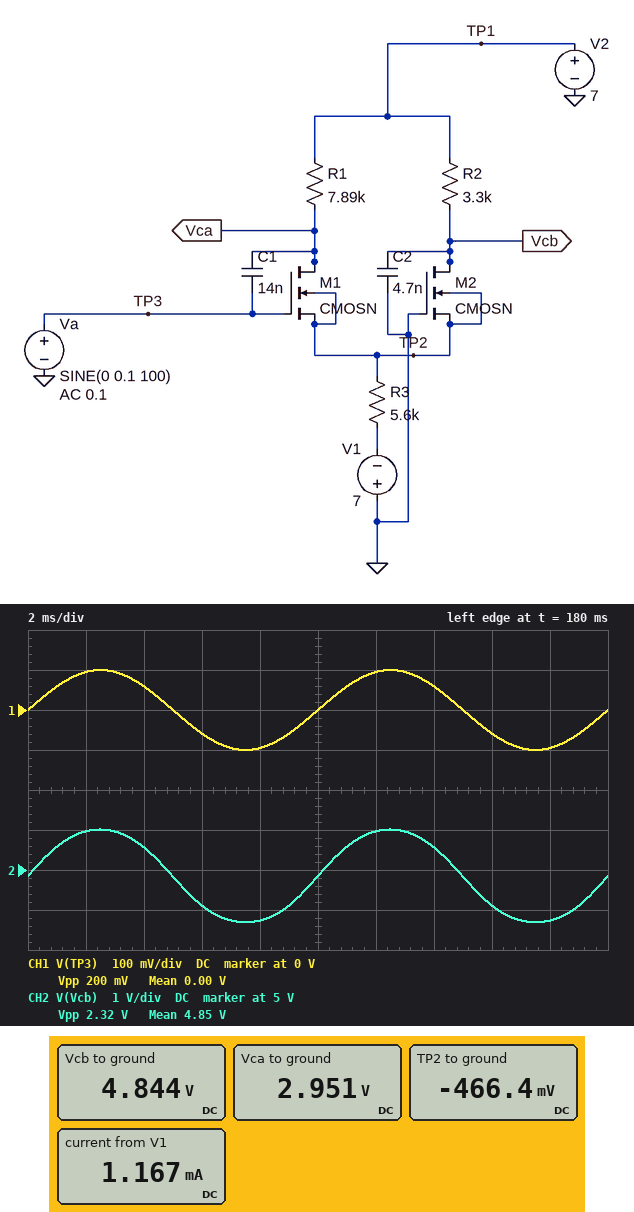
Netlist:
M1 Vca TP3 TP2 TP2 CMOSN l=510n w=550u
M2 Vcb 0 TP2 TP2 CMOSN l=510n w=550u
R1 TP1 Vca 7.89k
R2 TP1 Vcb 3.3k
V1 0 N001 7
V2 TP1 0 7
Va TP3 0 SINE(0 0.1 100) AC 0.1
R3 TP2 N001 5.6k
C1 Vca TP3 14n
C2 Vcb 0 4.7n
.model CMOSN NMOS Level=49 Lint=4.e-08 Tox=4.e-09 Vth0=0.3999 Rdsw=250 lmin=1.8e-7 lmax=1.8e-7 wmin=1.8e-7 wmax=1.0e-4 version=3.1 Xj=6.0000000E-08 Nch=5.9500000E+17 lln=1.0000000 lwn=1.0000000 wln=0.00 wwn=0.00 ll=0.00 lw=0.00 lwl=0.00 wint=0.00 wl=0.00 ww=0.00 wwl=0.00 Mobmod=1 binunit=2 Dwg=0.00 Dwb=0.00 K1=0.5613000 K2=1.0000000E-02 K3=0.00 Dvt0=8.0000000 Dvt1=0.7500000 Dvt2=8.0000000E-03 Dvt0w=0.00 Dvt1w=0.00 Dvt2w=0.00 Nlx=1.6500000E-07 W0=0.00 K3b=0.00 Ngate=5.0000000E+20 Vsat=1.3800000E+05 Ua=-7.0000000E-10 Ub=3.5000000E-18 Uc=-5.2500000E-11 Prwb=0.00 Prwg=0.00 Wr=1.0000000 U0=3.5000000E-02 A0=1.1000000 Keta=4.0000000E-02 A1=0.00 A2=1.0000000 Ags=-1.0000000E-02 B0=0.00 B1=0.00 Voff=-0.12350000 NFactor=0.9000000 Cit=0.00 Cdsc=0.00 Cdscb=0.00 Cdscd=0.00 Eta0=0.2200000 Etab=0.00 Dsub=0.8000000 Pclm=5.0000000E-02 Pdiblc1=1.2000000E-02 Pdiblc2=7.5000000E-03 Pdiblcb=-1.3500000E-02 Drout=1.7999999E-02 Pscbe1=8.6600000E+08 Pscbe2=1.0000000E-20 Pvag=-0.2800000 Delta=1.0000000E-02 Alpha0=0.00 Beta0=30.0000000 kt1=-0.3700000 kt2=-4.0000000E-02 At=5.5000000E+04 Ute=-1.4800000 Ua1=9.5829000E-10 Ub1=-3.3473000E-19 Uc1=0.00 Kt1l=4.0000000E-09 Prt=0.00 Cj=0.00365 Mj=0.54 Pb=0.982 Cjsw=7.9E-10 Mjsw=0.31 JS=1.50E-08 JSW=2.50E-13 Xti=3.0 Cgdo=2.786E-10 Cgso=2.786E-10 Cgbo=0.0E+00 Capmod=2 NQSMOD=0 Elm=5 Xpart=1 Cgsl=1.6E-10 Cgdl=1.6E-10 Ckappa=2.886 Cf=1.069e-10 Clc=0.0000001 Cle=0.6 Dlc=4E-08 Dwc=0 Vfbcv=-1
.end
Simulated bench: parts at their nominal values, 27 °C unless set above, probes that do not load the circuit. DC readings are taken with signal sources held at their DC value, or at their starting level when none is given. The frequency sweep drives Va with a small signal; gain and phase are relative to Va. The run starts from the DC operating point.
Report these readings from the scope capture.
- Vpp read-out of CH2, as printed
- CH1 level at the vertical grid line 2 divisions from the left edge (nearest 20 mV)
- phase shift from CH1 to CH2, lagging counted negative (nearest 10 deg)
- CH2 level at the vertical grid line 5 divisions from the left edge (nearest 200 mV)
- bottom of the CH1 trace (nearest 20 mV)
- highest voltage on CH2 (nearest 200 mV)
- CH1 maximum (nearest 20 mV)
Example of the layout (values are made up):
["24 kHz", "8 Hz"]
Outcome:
["2.32 V", "60 mV", "0 deg", "4.8 V", "-100 mV", "6.0 V", "100 mV"]
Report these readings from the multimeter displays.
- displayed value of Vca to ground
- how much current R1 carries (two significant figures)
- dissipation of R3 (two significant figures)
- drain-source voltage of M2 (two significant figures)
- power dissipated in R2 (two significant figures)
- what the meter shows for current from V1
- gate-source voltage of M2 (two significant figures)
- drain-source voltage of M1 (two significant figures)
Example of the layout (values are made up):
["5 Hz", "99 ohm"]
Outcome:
["2.951 V", "510 µA", "7.6 mW", "5.3 V", "1.4 mW", "1.167 mA", "470 mV", "3.4 V"]
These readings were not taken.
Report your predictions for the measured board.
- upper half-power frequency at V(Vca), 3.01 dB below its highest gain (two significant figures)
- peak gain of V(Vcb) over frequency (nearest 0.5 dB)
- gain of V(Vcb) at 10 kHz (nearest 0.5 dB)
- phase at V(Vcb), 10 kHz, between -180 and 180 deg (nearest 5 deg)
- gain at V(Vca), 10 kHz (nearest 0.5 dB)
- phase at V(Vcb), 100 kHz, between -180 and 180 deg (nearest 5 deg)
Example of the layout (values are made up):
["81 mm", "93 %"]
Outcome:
["1.9 kHz", "23.5 dB", "22.0 dB", "-40 deg", "15.5 dB", "-85 deg"]
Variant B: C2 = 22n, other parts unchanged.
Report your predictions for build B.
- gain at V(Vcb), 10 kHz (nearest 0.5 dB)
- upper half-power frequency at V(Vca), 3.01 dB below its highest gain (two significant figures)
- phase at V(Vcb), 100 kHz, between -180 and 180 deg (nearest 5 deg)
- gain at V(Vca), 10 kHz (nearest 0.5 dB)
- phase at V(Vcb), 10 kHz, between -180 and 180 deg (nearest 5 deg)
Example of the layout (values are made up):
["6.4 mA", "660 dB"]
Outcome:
["12.0 dB", "2.0 kHz", "-90 deg", "16.0 dB", "-75 deg"]
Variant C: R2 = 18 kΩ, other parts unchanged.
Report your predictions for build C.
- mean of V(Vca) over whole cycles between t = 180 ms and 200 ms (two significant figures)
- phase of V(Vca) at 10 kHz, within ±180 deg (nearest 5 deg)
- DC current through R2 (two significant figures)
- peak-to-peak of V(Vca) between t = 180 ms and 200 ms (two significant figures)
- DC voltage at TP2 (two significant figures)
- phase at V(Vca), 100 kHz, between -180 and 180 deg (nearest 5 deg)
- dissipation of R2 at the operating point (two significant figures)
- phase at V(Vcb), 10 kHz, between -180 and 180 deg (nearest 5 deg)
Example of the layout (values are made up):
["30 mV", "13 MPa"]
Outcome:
["750 mV", "70 deg", "410 µA", "1.6 V", "-500 mV", "35 deg", "3.1 mW", "-5 deg"]
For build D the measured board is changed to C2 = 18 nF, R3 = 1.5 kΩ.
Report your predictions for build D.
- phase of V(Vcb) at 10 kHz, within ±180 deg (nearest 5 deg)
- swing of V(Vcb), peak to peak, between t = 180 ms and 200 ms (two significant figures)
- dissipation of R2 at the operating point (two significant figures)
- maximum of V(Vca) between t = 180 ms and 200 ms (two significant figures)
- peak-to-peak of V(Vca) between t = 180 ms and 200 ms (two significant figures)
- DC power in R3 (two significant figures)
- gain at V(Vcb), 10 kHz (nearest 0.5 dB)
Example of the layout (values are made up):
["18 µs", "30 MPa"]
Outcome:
["30 deg", "1.6 mV", "22 mW", "-1.5 V", "1.7 mV", "20 mW", "-8.5 dB"]
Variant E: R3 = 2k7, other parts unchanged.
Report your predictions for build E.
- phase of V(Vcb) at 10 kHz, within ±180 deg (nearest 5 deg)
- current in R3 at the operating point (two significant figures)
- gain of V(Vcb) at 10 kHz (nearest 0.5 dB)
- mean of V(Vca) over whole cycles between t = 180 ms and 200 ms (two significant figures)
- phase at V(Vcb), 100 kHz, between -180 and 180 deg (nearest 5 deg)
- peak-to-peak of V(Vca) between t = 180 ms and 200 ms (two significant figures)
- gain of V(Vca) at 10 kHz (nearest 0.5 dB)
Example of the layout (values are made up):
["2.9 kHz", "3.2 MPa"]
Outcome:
["-30 deg", "2.4 mA", "25.0 dB", "680 mV", "-80 deg", "3.6 V", "18.5 dB"]
